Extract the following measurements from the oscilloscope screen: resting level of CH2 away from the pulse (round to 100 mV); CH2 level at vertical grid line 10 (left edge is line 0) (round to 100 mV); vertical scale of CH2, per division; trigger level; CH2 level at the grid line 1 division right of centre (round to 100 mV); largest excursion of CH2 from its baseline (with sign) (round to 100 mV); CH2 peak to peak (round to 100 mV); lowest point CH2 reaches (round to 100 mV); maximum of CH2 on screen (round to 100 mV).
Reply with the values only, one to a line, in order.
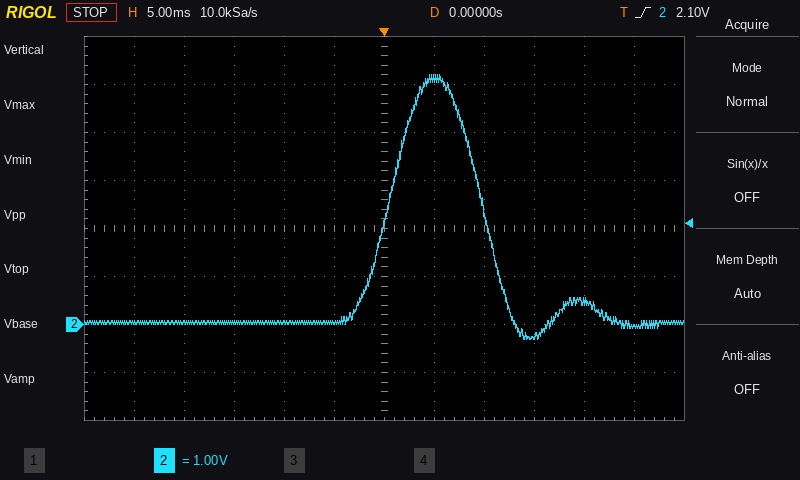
0.0 V
500 mV
1 V
2.10 V
5.1 V
+5.2 V
5.5 V
-300 mV
5.2 V
